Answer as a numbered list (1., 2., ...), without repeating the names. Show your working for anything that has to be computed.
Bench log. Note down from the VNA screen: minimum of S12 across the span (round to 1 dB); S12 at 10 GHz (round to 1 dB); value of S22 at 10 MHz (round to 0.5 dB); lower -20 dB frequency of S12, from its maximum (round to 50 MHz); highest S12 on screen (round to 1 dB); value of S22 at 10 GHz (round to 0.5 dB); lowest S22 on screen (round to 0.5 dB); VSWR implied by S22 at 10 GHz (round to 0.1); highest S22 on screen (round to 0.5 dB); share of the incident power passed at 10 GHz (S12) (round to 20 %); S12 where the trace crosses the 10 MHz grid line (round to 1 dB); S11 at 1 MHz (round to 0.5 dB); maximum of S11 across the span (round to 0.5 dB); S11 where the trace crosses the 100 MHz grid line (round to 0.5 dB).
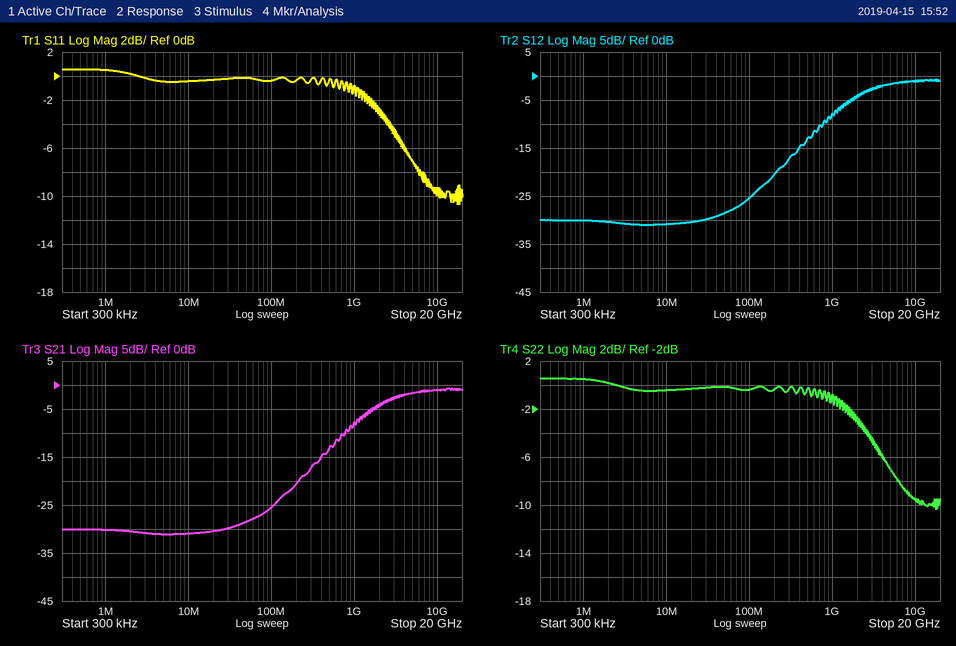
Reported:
1. -31 dB
2. -1 dB
3. -0.5 dB
4. 200 MHz
5. -1 dB
6. -9.5 dB
7. -10.5 dB
8. |Γ| = 10^(-9.5/20) = 0.3350; VSWR = (1 + 0.3350)/(1 − 0.3350) ≈ 2.0
9. 0.5 dB
10. 10^(-1/10) ≈ 79.4 %, so 80 % to the nearest 20 %
11. -31 dB
12. 0.5 dB
13. 0.5 dB
14. -0.5 dB
